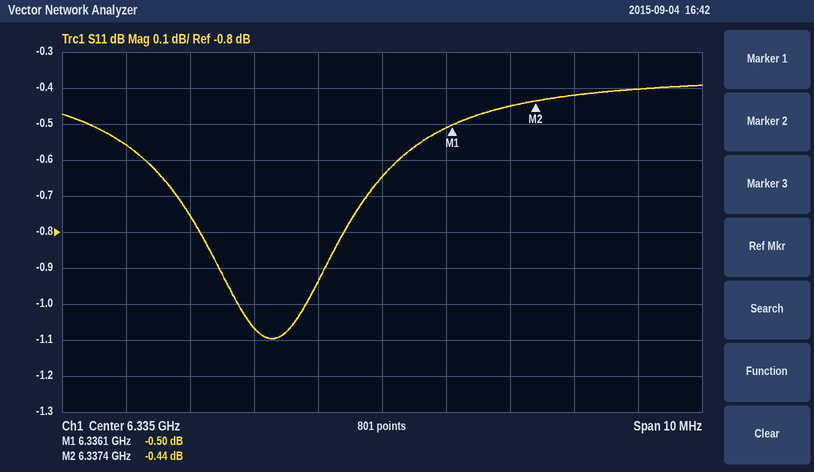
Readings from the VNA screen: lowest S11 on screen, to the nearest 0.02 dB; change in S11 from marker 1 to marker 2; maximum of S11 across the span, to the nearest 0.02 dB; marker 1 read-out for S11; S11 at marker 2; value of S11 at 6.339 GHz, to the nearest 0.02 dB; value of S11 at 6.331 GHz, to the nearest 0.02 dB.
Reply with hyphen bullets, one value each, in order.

- -1.10 dB
- 0.06 dB
- -0.40 dB
- -0.50 dB
- -0.44 dB
- -0.40 dB
- -0.56 dB
